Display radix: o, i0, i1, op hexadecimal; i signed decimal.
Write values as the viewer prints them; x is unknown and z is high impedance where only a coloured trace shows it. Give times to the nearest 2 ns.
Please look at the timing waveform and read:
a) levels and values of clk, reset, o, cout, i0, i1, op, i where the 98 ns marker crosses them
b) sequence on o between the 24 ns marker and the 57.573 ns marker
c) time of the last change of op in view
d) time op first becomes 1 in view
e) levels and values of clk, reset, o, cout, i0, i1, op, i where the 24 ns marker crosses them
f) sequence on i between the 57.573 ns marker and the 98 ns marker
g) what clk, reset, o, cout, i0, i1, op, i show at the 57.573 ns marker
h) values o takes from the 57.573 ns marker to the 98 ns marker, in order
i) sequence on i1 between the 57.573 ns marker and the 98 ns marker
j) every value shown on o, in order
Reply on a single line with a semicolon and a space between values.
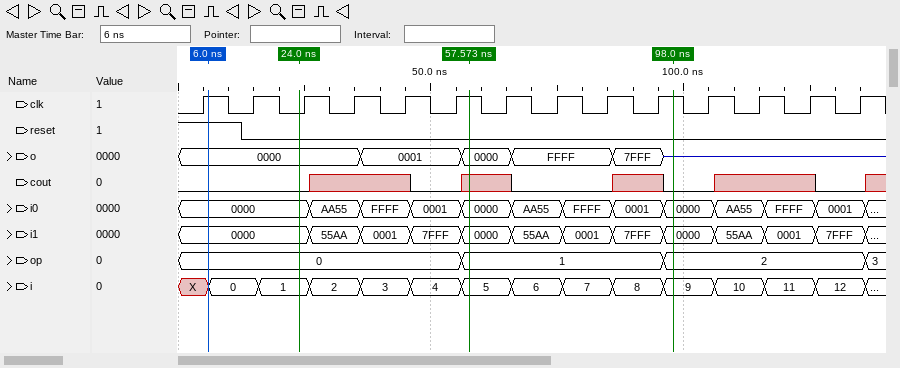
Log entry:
clk=1, reset=0, o=z, cout=0, i0=0000, i1=0000, op=2, i=9; 0000, 0001, 0000; 136 ns; 56 ns; clk=0, reset=0, o=0000, cout=0, i0=0000, i1=0000, op=0, i=1; 5, 6, 7, 8, 9; clk=1, reset=0, o=0000, cout=x, i0=0000, i1=0000, op=1, i=5; 0000, FFFF, 7FFF, z; 0000, 55AA, 0001, 7FFF, 0000; 0000, 0001, 0000, FFFF, 7FFF, z
